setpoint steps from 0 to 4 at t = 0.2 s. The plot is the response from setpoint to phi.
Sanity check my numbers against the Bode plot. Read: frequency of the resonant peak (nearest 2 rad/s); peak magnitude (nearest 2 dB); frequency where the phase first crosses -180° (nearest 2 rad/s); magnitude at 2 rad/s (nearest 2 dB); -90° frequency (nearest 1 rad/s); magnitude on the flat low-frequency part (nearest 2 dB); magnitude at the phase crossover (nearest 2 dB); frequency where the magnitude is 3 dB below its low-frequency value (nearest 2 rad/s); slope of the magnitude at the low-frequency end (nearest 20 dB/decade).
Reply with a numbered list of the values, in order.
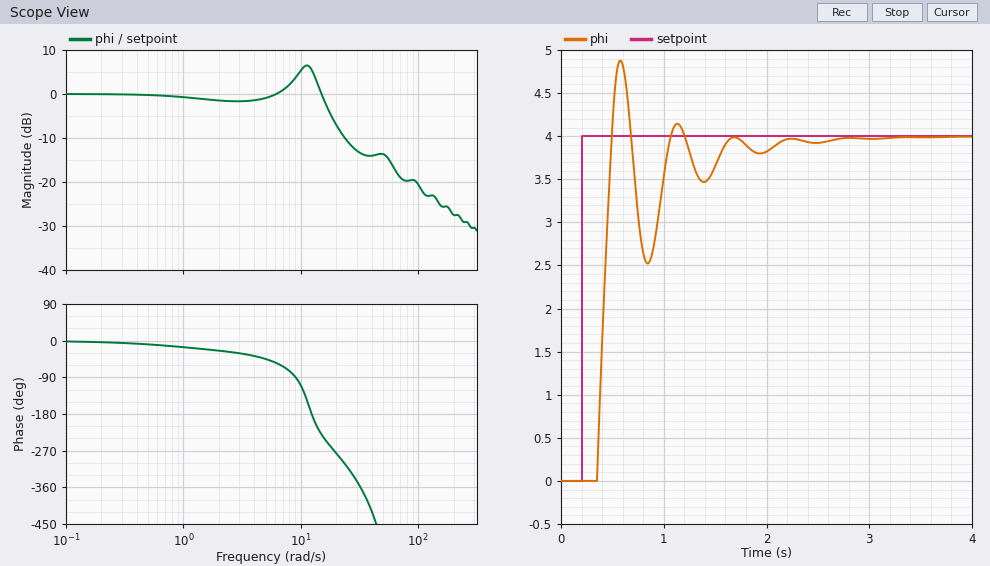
1. 12 rad/s
2. 6 dB
3. 12 rad/s
4. -2 dB
5. 9 rad/s
6. 0 dB
7. 6 dB
8. 16 rad/s
9. 0 dB/decade
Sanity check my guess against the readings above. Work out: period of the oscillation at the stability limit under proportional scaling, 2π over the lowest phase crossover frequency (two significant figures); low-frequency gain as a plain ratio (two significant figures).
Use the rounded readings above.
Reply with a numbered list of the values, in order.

1. 0.52 s
2. 1.0
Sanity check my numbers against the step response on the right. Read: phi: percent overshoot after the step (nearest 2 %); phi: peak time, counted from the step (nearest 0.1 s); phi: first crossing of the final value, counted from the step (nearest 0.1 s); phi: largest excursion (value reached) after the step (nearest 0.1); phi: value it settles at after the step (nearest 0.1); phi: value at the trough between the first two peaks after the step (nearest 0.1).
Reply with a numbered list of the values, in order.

1. 22 %
2. 0.4 s
3. 0.3 s
4. 4.9
5. 4.0
6. 2.5
